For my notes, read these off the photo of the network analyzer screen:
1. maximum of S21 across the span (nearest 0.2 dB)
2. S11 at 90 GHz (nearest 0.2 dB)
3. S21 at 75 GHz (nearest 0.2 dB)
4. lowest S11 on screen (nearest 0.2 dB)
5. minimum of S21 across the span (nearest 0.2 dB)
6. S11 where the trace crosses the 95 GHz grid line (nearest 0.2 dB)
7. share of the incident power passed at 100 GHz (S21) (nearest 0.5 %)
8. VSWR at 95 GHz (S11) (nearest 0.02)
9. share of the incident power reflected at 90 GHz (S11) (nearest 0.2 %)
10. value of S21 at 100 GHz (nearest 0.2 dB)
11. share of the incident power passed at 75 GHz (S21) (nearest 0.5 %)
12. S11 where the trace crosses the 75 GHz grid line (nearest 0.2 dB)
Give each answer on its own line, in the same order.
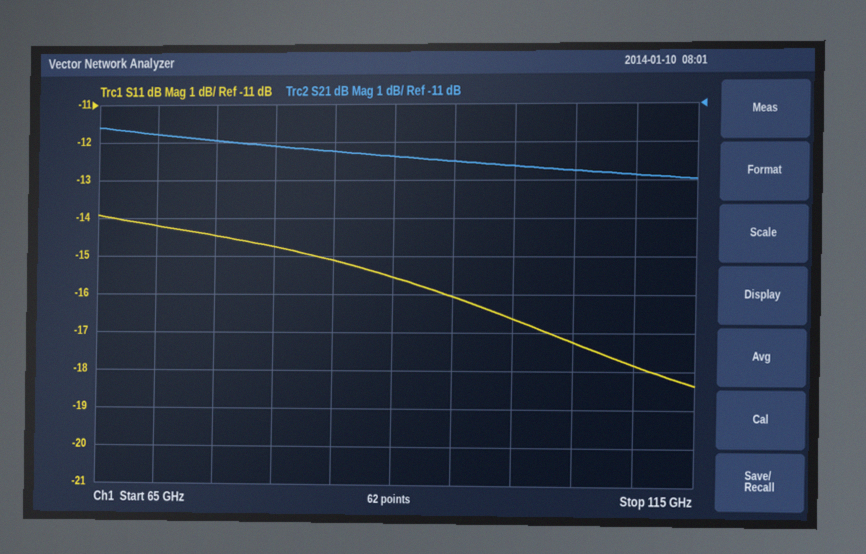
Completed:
-11.6 dB
-15.6 dB
-12.0 dB
-18.4 dB
-13.0 dB
-16.0 dB
5.5 %
1.38
2.8 %
-12.6 dB
6.5 %
-14.4 dB
